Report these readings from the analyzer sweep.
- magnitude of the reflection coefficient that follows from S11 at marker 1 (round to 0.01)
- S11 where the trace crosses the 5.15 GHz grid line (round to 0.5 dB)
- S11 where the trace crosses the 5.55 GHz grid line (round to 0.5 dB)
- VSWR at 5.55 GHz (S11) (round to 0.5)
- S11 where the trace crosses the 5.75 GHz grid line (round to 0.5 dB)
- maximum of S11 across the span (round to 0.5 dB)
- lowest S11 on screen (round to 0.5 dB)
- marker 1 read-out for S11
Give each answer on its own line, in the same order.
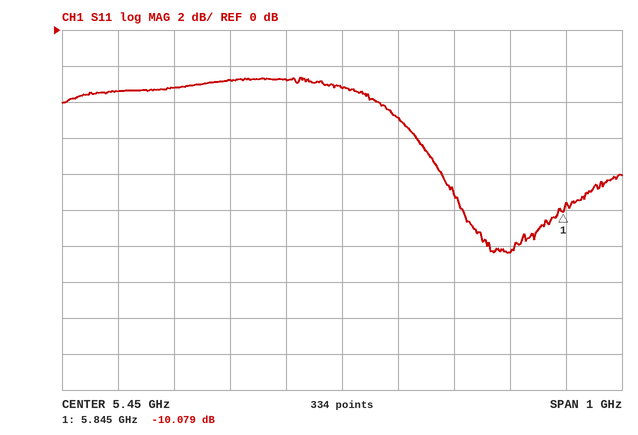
0.31
-3.0 dB
-5.0 dB
3.5
-12.5 dB
-2.5 dB
-12.5 dB
-10.079 dB
